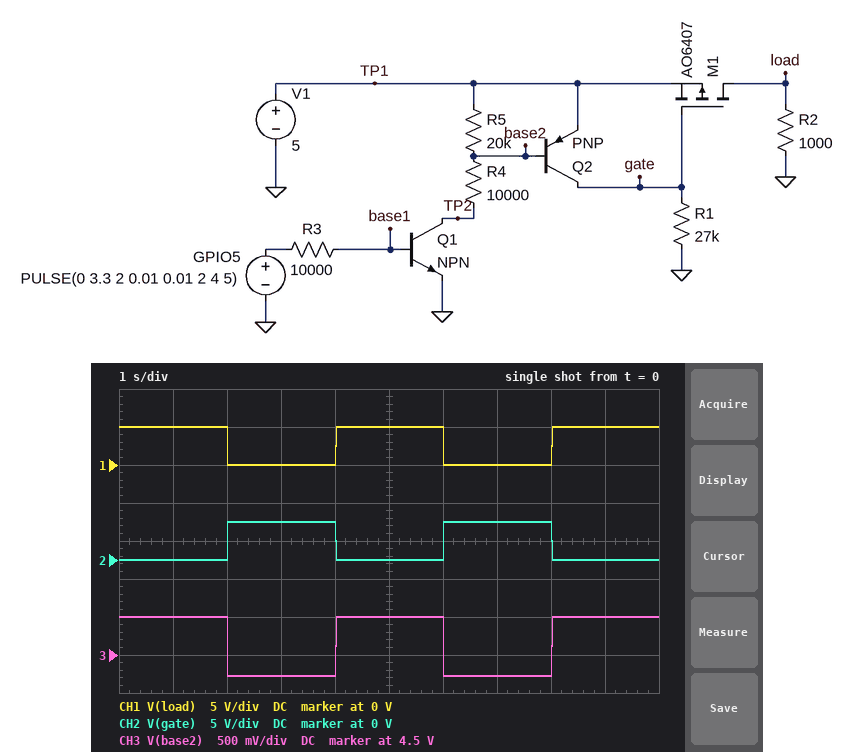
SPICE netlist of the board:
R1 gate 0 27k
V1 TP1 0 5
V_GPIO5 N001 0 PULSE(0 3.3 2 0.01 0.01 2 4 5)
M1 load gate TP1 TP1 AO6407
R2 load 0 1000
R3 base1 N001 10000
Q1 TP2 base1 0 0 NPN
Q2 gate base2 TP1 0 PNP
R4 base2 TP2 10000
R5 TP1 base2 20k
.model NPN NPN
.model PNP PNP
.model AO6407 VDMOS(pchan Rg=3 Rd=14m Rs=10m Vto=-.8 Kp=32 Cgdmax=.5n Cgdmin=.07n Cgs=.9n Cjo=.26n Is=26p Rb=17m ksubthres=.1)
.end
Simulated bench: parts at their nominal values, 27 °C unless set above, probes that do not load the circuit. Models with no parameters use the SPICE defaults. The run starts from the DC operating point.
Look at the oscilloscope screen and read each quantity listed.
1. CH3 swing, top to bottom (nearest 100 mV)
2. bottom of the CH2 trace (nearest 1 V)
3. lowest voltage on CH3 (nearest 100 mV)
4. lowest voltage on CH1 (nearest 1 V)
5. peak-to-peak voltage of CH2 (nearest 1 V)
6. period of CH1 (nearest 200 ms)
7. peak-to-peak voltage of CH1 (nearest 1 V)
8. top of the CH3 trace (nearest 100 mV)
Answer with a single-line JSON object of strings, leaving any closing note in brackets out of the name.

{"CH3 swing, top to bottom": "800 mV", "bottom of the CH2 trace": "0 V", "lowest voltage on CH3": "4.2 V", "lowest voltage on CH1": "0 V", "peak-to-peak voltage of CH2": "5 V", "period of CH1": "4.0 s", "peak-to-peak voltage of CH1": "5 V", "top of the CH3 trace": "5.0 V"}
